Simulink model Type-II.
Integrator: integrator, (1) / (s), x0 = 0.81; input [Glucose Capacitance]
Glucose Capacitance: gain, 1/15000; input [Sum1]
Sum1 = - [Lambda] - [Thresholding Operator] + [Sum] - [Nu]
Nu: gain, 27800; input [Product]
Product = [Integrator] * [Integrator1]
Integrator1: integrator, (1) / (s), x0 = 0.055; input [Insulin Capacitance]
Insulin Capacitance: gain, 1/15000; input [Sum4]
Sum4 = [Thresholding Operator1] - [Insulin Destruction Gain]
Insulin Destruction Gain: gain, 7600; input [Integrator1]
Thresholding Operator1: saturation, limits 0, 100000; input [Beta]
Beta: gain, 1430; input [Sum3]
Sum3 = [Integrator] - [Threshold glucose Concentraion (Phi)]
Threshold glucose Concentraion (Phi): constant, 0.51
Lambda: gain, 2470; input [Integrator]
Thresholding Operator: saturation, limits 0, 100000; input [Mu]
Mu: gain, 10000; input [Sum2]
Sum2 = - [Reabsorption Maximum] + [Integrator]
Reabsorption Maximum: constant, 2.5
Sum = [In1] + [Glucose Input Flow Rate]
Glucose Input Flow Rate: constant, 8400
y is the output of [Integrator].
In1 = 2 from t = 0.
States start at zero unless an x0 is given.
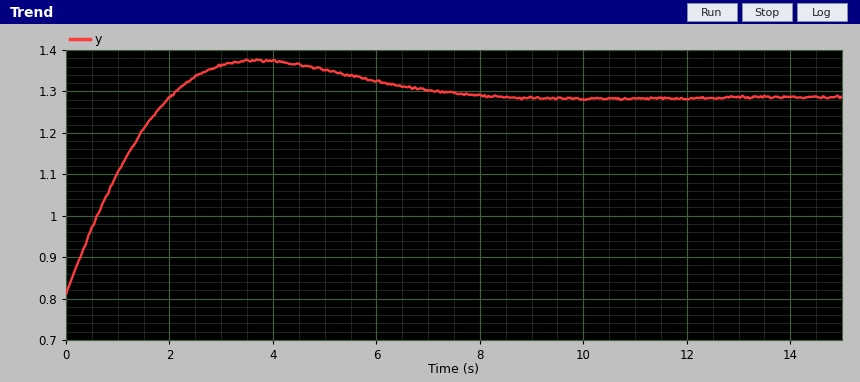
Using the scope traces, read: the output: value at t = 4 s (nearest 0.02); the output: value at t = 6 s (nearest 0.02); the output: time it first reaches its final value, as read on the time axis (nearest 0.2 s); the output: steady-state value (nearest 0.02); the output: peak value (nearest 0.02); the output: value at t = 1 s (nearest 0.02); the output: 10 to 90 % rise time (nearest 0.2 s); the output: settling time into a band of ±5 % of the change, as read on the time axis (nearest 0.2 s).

1.38
1.32
2.0 s
1.28
1.38
1.10
1.6 s
6.6 s
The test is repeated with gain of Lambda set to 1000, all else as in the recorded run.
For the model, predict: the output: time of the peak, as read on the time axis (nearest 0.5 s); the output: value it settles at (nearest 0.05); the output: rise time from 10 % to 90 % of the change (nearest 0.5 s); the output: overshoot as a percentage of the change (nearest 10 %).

3.5 s
1.45
1.5 s
20 %
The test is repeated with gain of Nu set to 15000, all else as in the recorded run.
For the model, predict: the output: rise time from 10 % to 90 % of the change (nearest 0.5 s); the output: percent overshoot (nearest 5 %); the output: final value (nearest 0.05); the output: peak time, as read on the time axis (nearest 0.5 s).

2.5 s
10 %
1.55
5.0 s
